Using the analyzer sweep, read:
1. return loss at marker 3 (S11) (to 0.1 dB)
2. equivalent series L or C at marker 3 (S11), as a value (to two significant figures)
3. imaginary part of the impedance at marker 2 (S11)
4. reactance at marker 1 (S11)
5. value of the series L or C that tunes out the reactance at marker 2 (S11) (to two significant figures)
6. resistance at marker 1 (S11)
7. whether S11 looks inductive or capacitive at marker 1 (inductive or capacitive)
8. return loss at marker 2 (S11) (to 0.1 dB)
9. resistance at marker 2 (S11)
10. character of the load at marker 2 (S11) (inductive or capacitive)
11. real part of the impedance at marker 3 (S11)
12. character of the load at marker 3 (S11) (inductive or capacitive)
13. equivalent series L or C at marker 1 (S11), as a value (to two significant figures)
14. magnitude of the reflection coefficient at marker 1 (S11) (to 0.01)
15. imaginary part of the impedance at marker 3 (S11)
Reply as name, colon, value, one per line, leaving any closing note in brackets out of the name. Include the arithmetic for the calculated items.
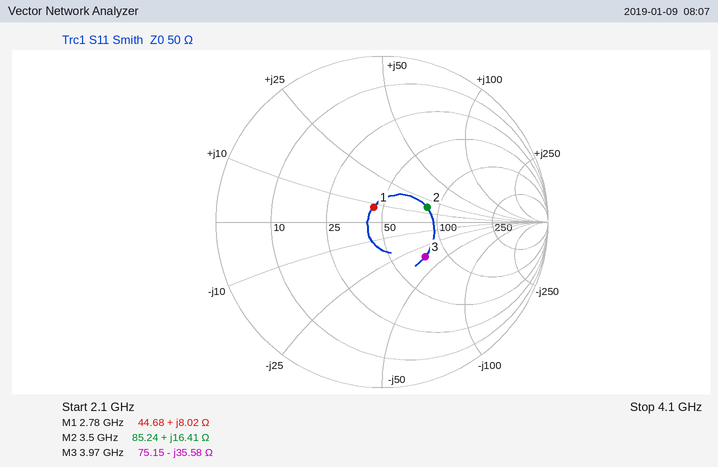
return loss at marker 3 (S11): 9.5 dB
equivalent series L or C at marker 3 (S11), as a value: C = 1/(2π × 3.97 GHz × 35.58 Ω) ≈ 1.1 pF
imaginary part of the impedance at marker 2: +16.41 Ω
reactance at marker 1: +8.02 Ω
value of the series L or C that tunes out the reactance at marker 2 (S11): C = 1/(2π × 3.5 GHz × 16.41 Ω) ≈ 2.8 pF
resistance at marker 1: 44.68 Ω
whether S11 looks inductive or capacitive at marker 1: inductive
return loss at marker 2 (S11): 10.9 dB
resistance at marker 2: 85.24 Ω
character of the load at marker 2 (S11): inductive
real part of the impedance at marker 3: 75.15 Ω
character of the load at marker 3 (S11): capacitive
equivalent series L or C at marker 1 (S11), as a value: L = 8.02 Ω/(2π × 2.78 GHz) ≈ 459 pH, so 460 pH to two significant figures
magnitude of the reflection coefficient at marker 1 (S11): 0.10
imaginary part of the impedance at marker 3: -35.58 Ω
